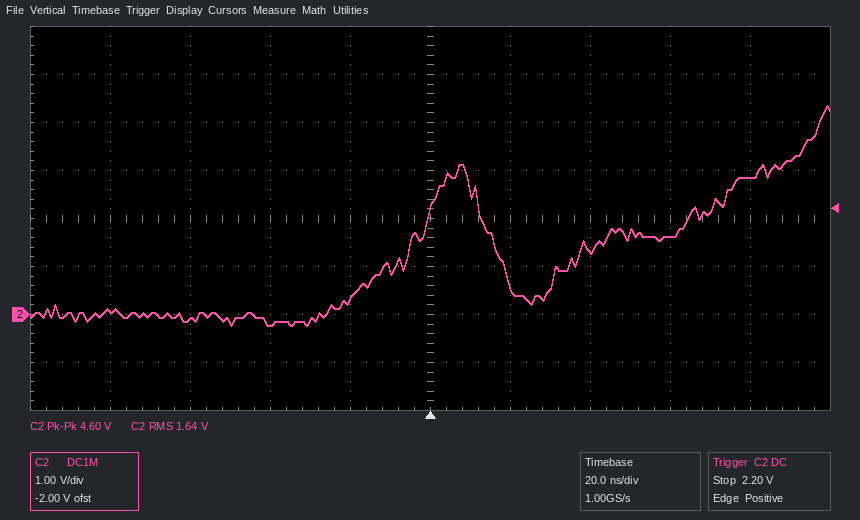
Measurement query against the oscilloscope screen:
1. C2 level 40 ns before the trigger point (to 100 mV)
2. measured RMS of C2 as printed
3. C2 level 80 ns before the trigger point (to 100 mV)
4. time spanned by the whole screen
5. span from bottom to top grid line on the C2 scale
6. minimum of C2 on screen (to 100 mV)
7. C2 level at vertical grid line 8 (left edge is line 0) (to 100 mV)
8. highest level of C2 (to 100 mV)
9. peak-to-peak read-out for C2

-200 mV
1.64 V
100 mV
200 ns
8 V
-200 mV
1.6 V
4.4 V
4.60 V
